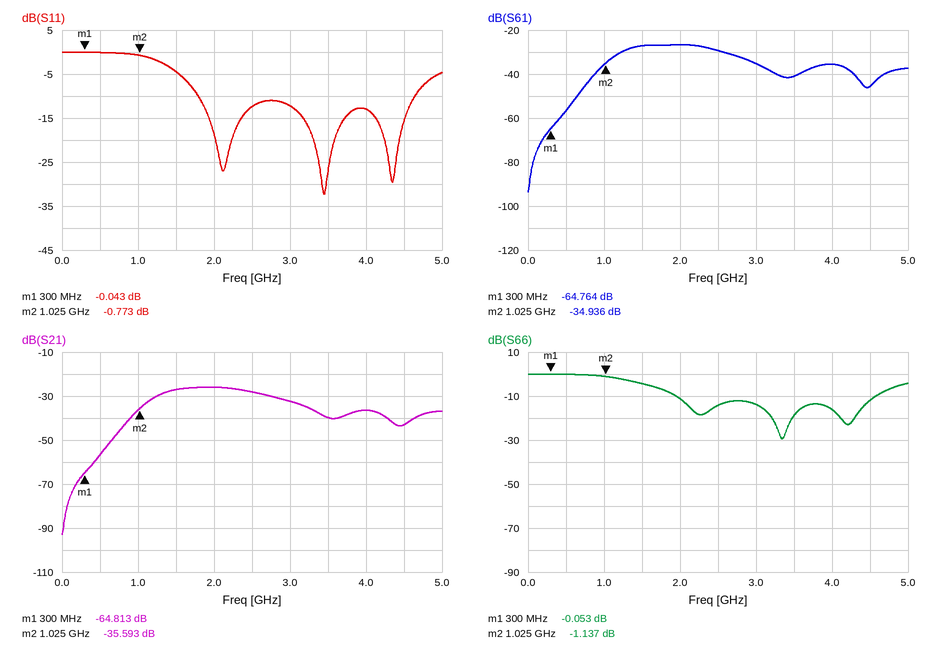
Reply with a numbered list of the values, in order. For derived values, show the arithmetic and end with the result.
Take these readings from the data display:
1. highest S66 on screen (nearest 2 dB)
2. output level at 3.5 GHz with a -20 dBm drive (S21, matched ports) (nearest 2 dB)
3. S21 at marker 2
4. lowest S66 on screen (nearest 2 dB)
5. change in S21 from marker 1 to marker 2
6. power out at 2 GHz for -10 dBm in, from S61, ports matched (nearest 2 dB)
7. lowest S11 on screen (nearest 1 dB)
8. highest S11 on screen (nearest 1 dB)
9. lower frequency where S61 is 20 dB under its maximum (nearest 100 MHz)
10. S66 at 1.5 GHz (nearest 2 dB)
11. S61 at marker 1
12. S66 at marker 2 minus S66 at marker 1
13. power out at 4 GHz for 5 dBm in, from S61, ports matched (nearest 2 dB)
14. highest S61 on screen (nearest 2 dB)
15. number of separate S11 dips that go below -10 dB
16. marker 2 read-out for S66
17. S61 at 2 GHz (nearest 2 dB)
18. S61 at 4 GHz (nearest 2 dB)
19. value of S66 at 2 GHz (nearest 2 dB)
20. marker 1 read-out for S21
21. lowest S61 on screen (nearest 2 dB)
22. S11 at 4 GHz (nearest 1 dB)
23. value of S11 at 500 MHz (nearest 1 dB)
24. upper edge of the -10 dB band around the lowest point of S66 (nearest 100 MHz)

1. 0 dB
2. -20 dBm + (-40 dB) = -60 dBm
3. -35.593 dB
4. -30 dB
5. -35.593 − (-64.813) = 29.220 dB
6. -10 dBm + (-26 dB) = -36 dBm
7. -32 dB
8. 0 dB
9. 700 MHz
10. -4 dB
11. -64.764 dB
12. -1.137 − (-0.053) = -1.084 dB
13. 5 dBm + (-36 dB) = -30 dBm
14. -26 dB
15. 3
16. -1.137 dB
17. -26 dB
18. -36 dB
19. -12 dB
20. -64.813 dB
21. -94 dB
22. -13 dB
23. 0 dB
24. 4.6 GHz
